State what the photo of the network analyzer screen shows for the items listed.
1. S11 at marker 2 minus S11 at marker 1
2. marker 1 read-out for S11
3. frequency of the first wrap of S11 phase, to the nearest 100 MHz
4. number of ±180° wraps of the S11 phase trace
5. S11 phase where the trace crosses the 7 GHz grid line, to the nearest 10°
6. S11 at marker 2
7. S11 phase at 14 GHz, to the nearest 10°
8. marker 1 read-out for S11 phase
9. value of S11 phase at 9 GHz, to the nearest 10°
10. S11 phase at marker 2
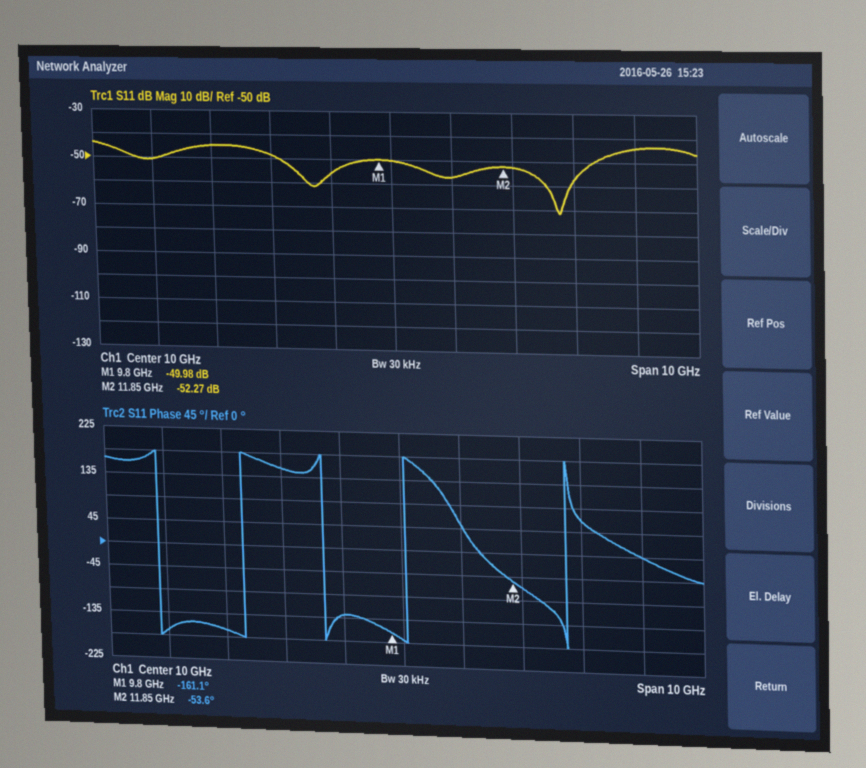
-2.29 dB
-49.98 dB
5.9 GHz
5
-170°
-52.27 dB
0°
-161.1°
-130°
-53.6°
